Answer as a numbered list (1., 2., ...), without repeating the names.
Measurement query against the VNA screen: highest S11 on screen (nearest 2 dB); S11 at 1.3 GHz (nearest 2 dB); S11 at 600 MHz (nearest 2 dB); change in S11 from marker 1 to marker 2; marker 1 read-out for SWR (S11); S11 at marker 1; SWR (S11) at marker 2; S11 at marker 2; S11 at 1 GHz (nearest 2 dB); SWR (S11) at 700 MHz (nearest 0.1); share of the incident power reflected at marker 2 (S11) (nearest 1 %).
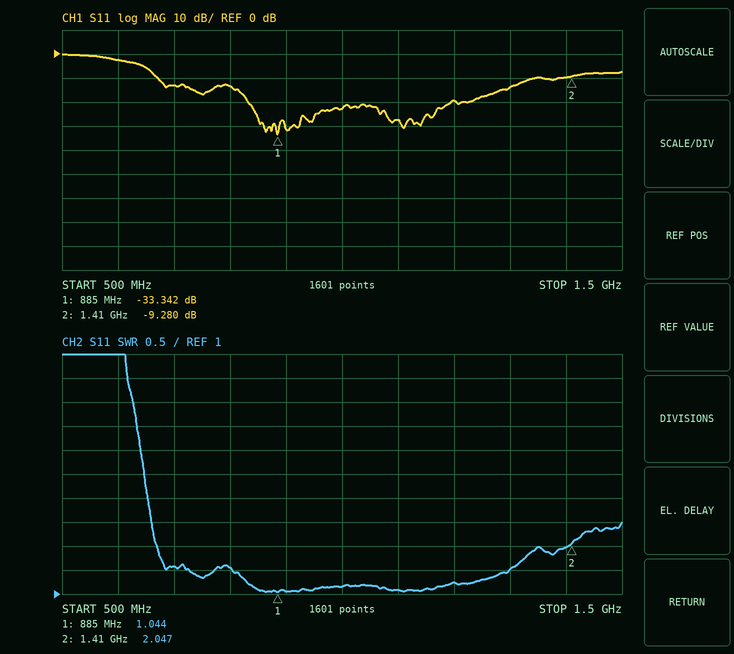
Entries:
1. 0 dB
2. -14 dB
3. -2 dB
4. 24.062 dB
5. 1.044
6. -33.342 dB
7. 2.047
8. -9.280 dB
9. -22 dB
10. 1.6
11. 12 %
